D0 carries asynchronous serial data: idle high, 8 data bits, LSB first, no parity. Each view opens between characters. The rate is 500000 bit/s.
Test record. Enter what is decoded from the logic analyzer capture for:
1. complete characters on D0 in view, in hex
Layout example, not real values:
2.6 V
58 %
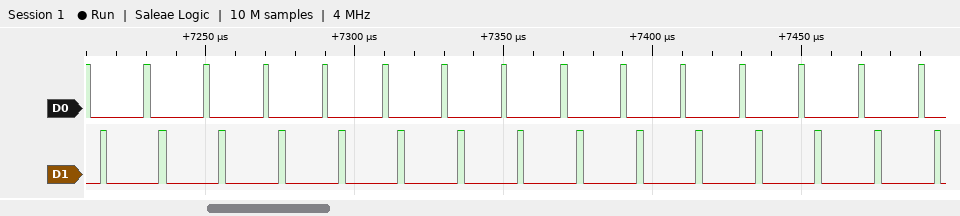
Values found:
00, 00, 00, 00, 00, 00, 00, 00, 00, 00, 00, 00, 00, 00
